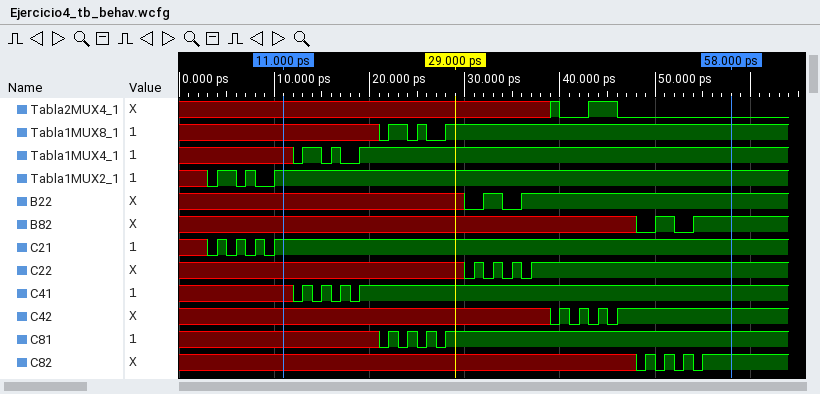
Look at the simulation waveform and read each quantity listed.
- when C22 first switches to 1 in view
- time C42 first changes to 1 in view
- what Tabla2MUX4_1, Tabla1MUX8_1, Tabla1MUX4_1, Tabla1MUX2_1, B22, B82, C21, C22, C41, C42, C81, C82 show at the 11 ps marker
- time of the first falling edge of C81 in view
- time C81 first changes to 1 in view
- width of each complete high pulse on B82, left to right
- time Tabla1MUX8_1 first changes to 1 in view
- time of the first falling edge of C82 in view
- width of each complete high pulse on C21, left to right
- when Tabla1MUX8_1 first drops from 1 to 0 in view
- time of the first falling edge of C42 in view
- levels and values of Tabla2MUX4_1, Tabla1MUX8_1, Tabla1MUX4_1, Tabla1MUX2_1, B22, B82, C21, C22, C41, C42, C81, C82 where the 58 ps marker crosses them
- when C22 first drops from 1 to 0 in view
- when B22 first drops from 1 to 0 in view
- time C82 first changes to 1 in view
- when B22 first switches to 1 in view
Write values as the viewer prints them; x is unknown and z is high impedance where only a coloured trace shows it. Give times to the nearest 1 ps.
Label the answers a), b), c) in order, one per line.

a) 31 ps
b) 40 ps
c) Tabla2MUX4_1=x, Tabla1MUX8_1=x, Tabla1MUX4_1=x, Tabla1MUX2_1=1, B22=x, B82=x, C21=1, C22=x, C41=x, C42=x, C81=x, C82=x
d) 23 ps
e) 22 ps
f) 2 ps
g) 22 ps
h) 50 ps
i) 1 ps, 1 ps, 1 ps
j) 24 ps
k) 41 ps
l) Tabla2MUX4_1=0, Tabla1MUX8_1=1, Tabla1MUX4_1=1, Tabla1MUX2_1=1, B22=1, B82=1, C21=1, C22=1, C41=1, C42=1, C81=1, C82=1
m) 32 ps
n) 34 ps
o) 49 ps
p) 32 ps
